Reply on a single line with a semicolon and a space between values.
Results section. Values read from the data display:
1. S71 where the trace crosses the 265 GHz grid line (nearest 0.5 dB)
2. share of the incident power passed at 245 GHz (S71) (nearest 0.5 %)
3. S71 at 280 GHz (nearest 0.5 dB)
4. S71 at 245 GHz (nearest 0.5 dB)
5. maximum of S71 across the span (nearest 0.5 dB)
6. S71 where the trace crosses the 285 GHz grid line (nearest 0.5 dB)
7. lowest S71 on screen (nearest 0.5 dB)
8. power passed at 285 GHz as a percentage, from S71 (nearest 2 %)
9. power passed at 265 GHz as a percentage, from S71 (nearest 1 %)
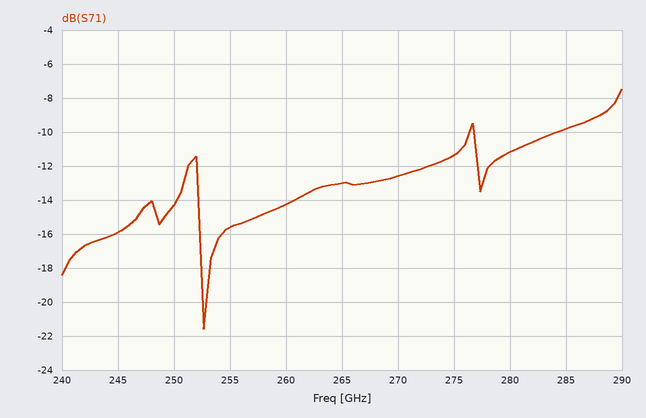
-13.0 dB; 2.5 %; -11.0 dB; -16.0 dB; -7.5 dB; -10.0 dB; -21.5 dB; 10 %; 5 %
